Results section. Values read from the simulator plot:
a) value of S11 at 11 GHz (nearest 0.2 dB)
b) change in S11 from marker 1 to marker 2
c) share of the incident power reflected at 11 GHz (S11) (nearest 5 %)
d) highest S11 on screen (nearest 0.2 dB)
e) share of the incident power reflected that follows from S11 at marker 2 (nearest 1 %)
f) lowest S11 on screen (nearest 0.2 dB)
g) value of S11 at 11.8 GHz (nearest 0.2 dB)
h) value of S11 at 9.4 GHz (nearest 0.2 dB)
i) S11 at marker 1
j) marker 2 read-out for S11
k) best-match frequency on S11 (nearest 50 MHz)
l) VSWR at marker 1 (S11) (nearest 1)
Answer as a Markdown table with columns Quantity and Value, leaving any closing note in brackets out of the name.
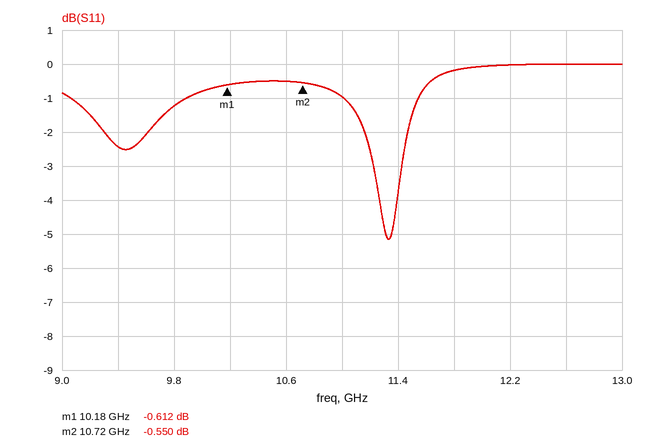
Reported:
| Quantity | Value |
|---|---|
| value of S11 at 11 GHz | -1.0 dB |
| change in S11 from marker 1 to marker 2 | 0.062 dB |
| share of the incident power reflected at 11 GHz (S11) | 80 % |
| highest S11 on screen | 0.0 dB |
| share of the incident power reflected that follows from S11 at marker 2 | 88 % |
| lowest S11 on screen | -5.2 dB |
| value of S11 at 11.8 GHz | -0.2 dB |
| value of S11 at 9.4 GHz | -2.4 dB |
| S11 at marker 1 | -0.612 dB |
| marker 2 read-out for S11 | -0.550 dB |
| best-match frequency on S11 | 11.35 GHz |
| VSWR at marker 1 (S11) | 28 |
